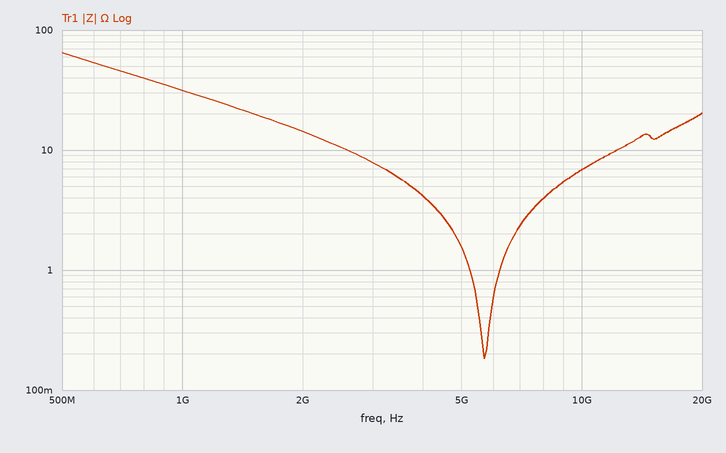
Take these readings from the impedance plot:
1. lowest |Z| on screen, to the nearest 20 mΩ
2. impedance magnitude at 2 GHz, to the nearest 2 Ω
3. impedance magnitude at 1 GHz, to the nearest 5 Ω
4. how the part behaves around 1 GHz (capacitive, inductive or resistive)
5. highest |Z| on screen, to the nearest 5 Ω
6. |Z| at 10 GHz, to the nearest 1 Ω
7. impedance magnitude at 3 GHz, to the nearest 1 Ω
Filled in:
180 mΩ
14 Ω
30 Ω
capacitive
65 Ω
7 Ω
8 Ω
